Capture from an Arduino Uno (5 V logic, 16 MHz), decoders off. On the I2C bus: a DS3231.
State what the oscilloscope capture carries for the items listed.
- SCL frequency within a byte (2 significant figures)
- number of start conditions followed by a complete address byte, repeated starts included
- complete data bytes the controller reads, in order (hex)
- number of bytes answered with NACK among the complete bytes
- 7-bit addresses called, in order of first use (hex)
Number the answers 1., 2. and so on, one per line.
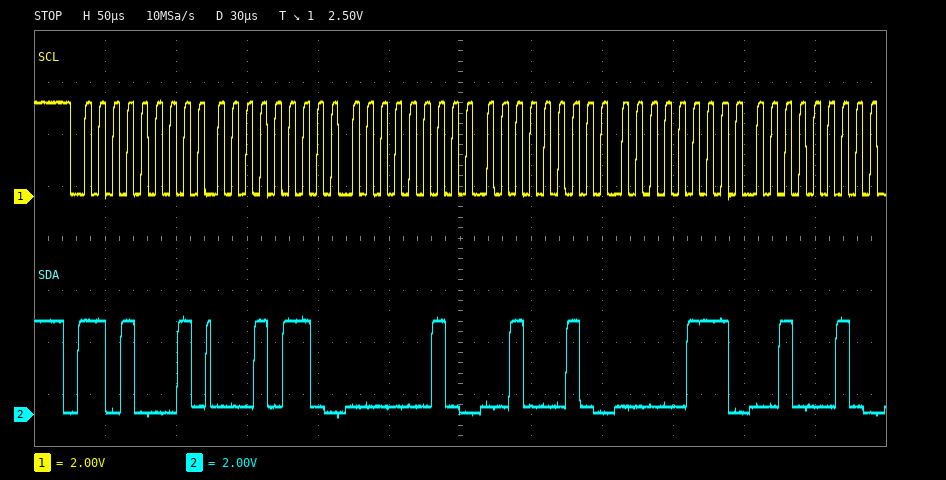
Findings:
1. 100 kHz
2. 1
3. 16 02 22 07 22
4. 0
5. 0x68
